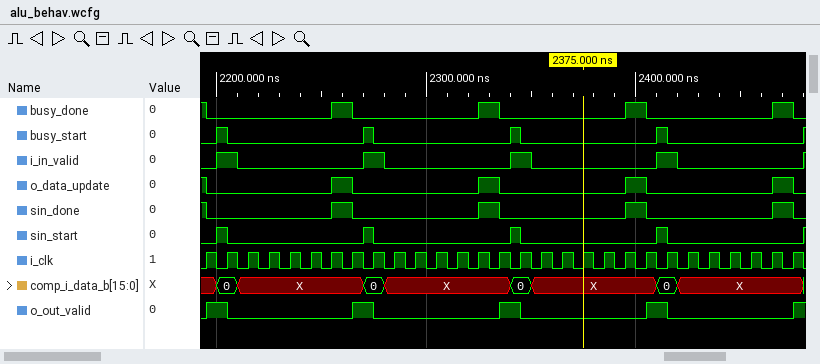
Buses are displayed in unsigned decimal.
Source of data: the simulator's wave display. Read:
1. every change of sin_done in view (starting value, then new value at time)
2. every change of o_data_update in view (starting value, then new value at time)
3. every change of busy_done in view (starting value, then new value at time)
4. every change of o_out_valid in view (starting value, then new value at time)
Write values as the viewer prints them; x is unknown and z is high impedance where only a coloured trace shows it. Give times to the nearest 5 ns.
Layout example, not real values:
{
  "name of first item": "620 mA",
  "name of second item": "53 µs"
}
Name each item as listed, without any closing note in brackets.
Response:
{
  "every change of sin_done in view": "1, 0 at 2195 ns, 1 at 2255 ns, 0 at 2265 ns, 1 at 2325 ns, 0 at 2335 ns, 1 at 2395 ns, 0 at 2405 ns, 1 at 2465 ns, 0 at 2475 ns",
  "every change of o_data_update in view": "1, 0 at 2195 ns, 1 at 2255 ns, 0 at 2265 ns, 1 at 2325 ns, 0 at 2335 ns, 1 at 2395 ns, 0 at 2405 ns, 1 at 2465 ns, 0 at 2475 ns",
  "every change of busy_done in view": "1, 0 at 2195 ns, 1 at 2255 ns, 0 at 2265 ns, 1 at 2325 ns, 0 at 2335 ns, 1 at 2395 ns, 0 at 2405 ns, 1 at 2465 ns, 0 at 2475 ns",
  "every change of o_out_valid in view": "0, 1 at 2195 ns, 0 at 2205 ns, 1 at 2265 ns, 0 at 2275 ns, 1 at 2335 ns, 0 at 2345 ns, 1 at 2405 ns, 0 at 2415 ns, 1 at 2475 ns"
}
